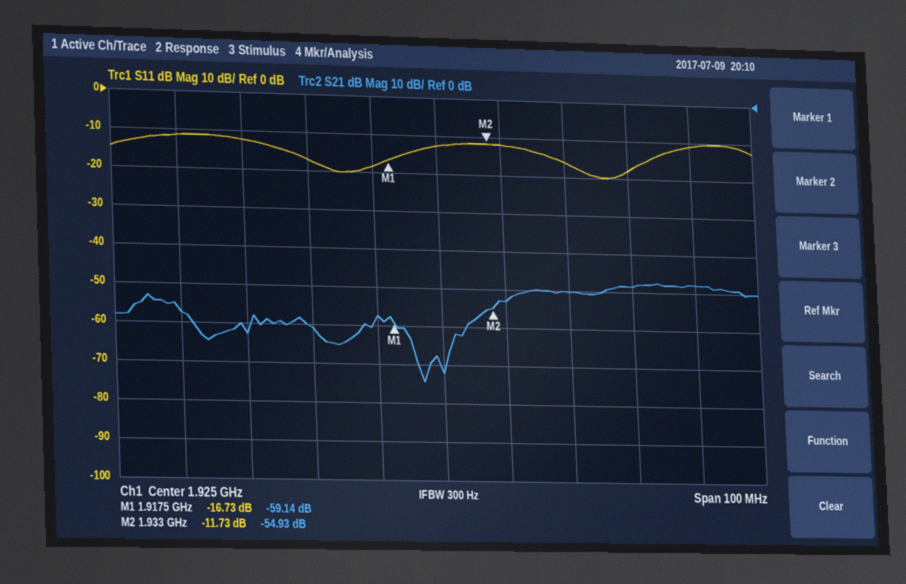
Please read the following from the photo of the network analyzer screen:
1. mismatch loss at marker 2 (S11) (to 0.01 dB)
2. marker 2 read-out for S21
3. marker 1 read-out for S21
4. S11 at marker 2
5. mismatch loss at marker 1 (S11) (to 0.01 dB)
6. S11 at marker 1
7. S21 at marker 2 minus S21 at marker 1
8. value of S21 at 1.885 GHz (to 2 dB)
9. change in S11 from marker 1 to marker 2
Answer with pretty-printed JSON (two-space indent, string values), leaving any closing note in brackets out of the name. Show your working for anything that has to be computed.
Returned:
{
  "mismatch loss at marker 2 (S11)": "−10 log10(1 − 10^(-11.73/10)) ≈ 0.30 dB",
  "marker 2 read-out for S21": "-54.93 dB",
  "marker 1 read-out for S21": "-59.14 dB",
  "S11 at marker 2": "-11.73 dB",
  "mismatch loss at marker 1 (S11)": "−10 log10(1 − 10^(-16.73/10)) ≈ 0.09 dB",
  "S11 at marker 1": "-16.73 dB",
  "S21 at marker 2 minus S21 at marker 1": "-54.93 − (-59.14) = 4.21 dB",
  "value of S21 at 1.885 GHz": "-58 dB",
  "change in S11 from marker 1 to marker 2": "-11.73 − (-16.73) = 5.00 dB"
}
